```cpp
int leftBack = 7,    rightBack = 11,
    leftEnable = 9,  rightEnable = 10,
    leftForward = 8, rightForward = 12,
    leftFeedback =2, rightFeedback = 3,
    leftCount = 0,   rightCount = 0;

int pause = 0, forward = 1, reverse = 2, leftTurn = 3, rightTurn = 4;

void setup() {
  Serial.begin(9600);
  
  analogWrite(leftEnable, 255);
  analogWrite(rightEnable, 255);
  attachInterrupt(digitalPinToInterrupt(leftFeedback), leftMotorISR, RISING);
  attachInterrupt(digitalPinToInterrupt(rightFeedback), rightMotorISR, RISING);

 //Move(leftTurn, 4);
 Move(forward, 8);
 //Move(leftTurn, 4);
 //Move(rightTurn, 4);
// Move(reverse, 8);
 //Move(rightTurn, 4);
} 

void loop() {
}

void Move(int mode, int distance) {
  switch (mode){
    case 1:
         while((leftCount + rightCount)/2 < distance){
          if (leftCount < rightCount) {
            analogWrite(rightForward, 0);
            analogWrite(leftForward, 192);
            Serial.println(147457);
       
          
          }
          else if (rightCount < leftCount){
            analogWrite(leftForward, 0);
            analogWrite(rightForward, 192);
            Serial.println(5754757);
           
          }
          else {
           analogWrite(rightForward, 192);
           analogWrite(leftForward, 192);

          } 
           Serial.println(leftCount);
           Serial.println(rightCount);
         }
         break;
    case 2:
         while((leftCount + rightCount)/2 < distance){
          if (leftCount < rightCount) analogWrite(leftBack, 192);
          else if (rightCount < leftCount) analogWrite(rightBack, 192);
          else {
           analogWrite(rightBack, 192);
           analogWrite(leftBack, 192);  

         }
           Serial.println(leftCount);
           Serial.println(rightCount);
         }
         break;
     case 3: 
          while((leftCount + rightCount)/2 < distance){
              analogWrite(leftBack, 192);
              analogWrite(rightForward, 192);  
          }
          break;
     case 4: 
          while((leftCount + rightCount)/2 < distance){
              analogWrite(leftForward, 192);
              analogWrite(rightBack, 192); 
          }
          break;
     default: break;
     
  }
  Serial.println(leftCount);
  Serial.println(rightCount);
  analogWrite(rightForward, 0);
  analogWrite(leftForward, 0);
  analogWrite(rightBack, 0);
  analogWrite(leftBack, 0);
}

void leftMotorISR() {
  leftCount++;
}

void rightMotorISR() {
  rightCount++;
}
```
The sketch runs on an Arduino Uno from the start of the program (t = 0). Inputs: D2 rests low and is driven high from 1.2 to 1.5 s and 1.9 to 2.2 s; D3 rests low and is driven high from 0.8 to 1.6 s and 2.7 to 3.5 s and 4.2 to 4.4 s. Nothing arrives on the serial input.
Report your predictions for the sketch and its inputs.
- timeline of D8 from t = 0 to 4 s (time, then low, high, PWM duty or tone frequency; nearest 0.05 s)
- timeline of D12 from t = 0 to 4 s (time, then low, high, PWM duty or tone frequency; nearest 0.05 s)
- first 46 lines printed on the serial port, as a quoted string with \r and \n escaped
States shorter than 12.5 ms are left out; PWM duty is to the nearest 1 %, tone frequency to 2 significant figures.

0 s high; 1.9 s low; 2.7 s high
0 s high; 0.8 s low; 1.2 s high
"0\r\n0\r\n0\r\n0\r\n0\r\n0\r\n0\r\n0\r\n0\r\n0\r\n0\r\n0\r\n0\r\n0\r\n0\r\n0\r\n0\r\n0\r\n0\r\n0\r\n0\r\n0\r\n0\r\n0\r\n0\r\n0\r\n0\r\n0\r\n0\r\n0\r\n0\r\n0\r\n0\r\n0\r\n0\r\n0\r\n0\r\n0\r\n0\r\n0\r\n0\r\n0\r\n0\r\n0\r\n0\r\n0\r\n"
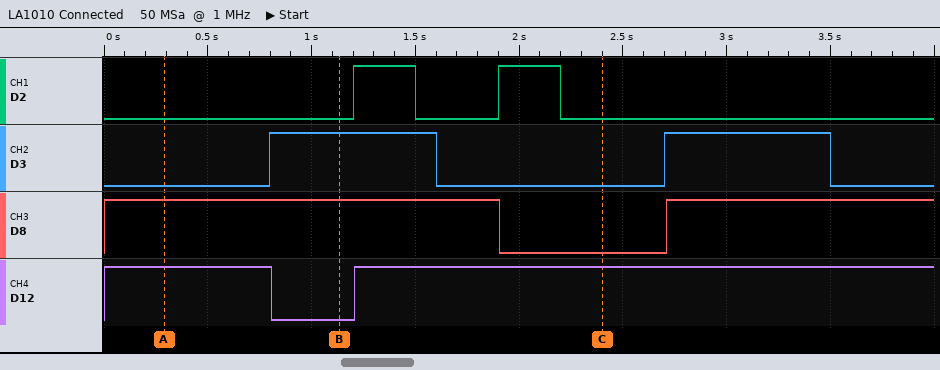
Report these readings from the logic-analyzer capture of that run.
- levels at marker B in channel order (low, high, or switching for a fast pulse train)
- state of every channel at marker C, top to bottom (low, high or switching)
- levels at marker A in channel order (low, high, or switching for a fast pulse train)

D2 low, D3 high, D8 high, D12 low
D2 low, D3 low, D8 low, D12 high
D2 low, D3 low, D8 high, D12 high
